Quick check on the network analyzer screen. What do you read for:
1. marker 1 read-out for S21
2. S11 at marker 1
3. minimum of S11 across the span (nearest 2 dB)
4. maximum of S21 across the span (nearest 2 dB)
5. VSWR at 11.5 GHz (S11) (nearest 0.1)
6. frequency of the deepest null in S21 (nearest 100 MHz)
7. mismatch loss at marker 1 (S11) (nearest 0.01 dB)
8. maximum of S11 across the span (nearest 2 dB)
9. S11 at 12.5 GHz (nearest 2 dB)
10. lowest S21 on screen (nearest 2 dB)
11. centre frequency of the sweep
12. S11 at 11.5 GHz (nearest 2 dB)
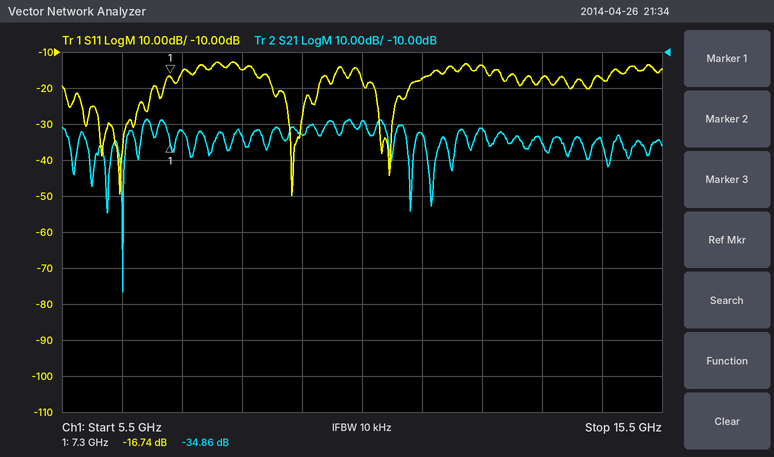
-34.86 dB
-16.74 dB
-50 dB
-28 dB
1.3
6.5 GHz
0.09 dB
-12 dB
-14 dB
-76 dB
10.5 GHz
-18 dB
